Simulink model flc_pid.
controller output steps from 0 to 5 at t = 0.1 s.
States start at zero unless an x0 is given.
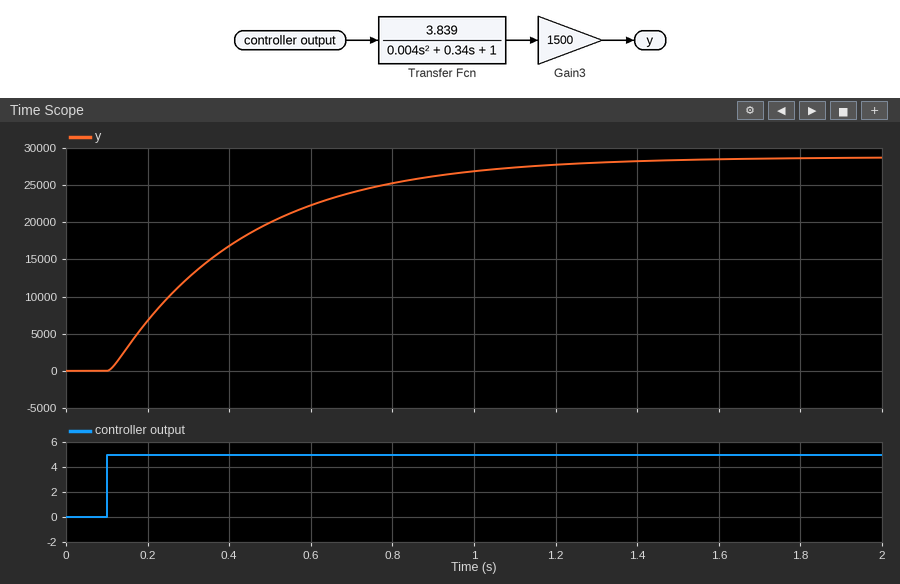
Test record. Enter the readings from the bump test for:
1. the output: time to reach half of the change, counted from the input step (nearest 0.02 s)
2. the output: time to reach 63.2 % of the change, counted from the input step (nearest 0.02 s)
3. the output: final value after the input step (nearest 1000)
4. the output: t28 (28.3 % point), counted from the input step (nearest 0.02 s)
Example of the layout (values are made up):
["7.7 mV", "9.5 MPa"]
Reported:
["0.24 s", "0.34 s", "29000", "0.12 s"]
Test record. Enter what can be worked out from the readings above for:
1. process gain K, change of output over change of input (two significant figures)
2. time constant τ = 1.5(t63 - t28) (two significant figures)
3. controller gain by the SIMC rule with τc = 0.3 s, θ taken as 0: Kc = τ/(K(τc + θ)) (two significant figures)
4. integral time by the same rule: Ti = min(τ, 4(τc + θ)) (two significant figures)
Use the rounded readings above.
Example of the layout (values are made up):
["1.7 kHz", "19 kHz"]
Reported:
["5800", "0.33 s", "0.00019", "0.33 s"]
